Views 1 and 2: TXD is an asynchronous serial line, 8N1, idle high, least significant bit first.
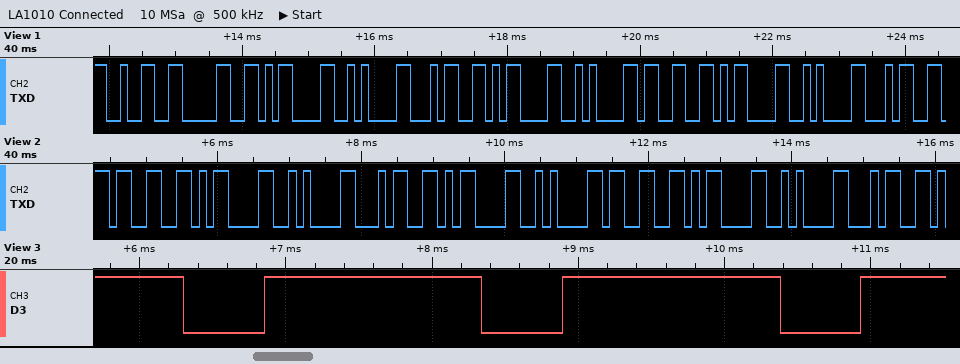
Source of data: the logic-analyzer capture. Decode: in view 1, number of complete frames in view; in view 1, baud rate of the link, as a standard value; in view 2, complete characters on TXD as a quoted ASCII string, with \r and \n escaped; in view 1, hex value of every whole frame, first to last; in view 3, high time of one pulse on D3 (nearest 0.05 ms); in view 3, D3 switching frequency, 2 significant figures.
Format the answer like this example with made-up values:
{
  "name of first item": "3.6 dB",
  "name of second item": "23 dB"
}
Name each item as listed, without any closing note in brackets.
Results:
{
  "in view 1, number of complete frames in view": "11",
  "in view 1, baud rate of the link, as a standard value": "9600 baud",
  "in view 2, complete characters on TXD as a quoted ASCII string, with \\r and \\n escaped": "\"3\\r\\n4\\r\\n3\\r\\n4\"",
  "in view 1, hex value of every whole frame, first to last": "32 30 0D 0A 34 0D 0A 33 0D 0A 34",
  "in view 3, high time of one pulse on D3": "1.50 ms",
  "in view 3, D3 switching frequency, 2 significant figures": "490 Hz"
}
